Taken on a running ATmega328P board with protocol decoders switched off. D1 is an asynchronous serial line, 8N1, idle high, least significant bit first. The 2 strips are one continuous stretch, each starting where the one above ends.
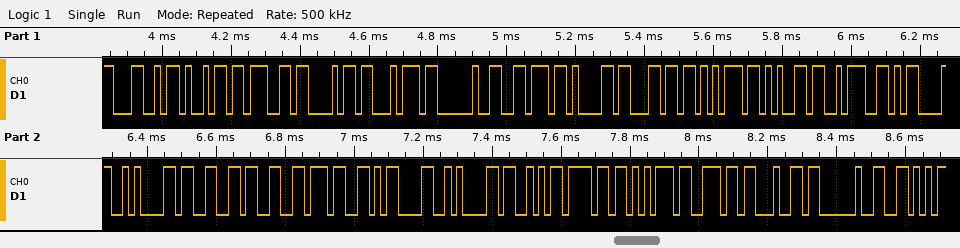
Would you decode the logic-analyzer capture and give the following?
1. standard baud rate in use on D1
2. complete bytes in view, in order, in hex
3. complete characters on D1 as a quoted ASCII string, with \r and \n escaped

57600 baud
4C 69 67 68 74 20 76 61 6C 75 65 3A 0D 0A 33 33 37 0D 0A 53 6F 75 6E 64 20 56
"Light value:\r\n337\r\nSound V"
